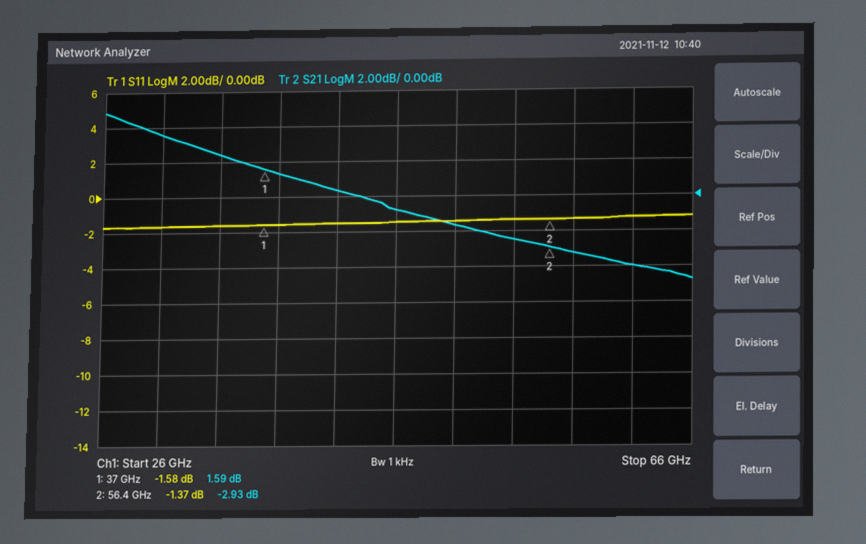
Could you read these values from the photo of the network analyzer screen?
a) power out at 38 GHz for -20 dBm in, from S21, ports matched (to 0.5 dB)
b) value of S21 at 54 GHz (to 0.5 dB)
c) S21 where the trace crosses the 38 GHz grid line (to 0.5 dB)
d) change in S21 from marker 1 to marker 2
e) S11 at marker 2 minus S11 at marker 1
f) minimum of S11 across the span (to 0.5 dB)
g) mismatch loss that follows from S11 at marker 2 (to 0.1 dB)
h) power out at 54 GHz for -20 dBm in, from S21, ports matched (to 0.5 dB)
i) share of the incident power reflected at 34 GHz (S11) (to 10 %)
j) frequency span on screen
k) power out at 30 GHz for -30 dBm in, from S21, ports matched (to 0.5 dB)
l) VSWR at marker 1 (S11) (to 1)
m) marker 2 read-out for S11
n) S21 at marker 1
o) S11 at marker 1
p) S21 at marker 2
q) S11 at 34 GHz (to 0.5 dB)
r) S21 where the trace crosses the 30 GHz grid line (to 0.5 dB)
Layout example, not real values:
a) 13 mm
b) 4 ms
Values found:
a) -18.5 dBm
b) -2.5 dB
c) 1.5 dB
d) -4.52 dB
e) 0.21 dB
f) -1.5 dB
g) 5.7 dB
h) -22.5 dBm
i) 70 %
j) 40 GHz
k) -26.5 dBm
l) 11
m) -1.37 dB
n) 1.59 dB
o) -1.58 dB
p) -2.93 dB
q) -1.5 dB
r) 3.5 dB
